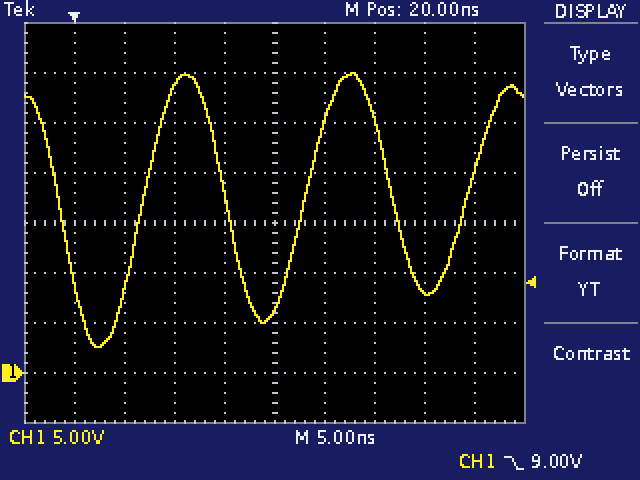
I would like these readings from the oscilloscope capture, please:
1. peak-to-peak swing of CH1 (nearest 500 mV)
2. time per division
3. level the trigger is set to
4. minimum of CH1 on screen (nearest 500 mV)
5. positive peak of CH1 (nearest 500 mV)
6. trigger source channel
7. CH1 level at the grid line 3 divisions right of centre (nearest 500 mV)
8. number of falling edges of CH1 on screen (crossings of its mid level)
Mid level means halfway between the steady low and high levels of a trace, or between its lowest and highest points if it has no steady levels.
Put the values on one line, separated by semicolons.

27.5 V; 5 ns; 9.00 V; 2.5 V; 30.0 V; CH1; 8.0 V; 3
